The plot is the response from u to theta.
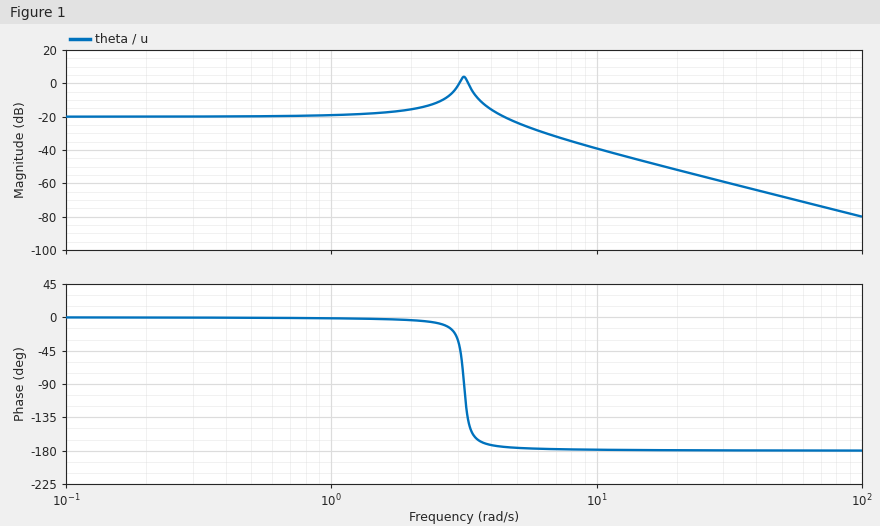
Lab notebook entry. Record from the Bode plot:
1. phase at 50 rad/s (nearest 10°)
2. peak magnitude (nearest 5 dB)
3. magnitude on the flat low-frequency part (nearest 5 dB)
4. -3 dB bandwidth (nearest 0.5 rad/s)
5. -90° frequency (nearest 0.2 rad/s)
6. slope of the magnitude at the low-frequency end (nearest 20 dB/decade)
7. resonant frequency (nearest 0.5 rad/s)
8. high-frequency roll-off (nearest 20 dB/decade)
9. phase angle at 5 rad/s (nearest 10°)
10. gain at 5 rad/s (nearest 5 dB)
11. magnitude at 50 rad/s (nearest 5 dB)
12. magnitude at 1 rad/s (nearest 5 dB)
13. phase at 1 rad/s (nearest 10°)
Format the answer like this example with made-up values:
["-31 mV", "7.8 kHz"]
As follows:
["-180°", "5 dB", "-20 dB", "5.0 rad/s", "3.2 rad/s", "0 dB/decade", "3.0 rad/s", "-40 dB/decade", "-180°", "-25 dB", "-70 dB", "-20 dB", "0°"]
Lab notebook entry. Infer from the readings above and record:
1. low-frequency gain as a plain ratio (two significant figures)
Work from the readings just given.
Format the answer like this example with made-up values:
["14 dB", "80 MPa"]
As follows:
["0.10"]
